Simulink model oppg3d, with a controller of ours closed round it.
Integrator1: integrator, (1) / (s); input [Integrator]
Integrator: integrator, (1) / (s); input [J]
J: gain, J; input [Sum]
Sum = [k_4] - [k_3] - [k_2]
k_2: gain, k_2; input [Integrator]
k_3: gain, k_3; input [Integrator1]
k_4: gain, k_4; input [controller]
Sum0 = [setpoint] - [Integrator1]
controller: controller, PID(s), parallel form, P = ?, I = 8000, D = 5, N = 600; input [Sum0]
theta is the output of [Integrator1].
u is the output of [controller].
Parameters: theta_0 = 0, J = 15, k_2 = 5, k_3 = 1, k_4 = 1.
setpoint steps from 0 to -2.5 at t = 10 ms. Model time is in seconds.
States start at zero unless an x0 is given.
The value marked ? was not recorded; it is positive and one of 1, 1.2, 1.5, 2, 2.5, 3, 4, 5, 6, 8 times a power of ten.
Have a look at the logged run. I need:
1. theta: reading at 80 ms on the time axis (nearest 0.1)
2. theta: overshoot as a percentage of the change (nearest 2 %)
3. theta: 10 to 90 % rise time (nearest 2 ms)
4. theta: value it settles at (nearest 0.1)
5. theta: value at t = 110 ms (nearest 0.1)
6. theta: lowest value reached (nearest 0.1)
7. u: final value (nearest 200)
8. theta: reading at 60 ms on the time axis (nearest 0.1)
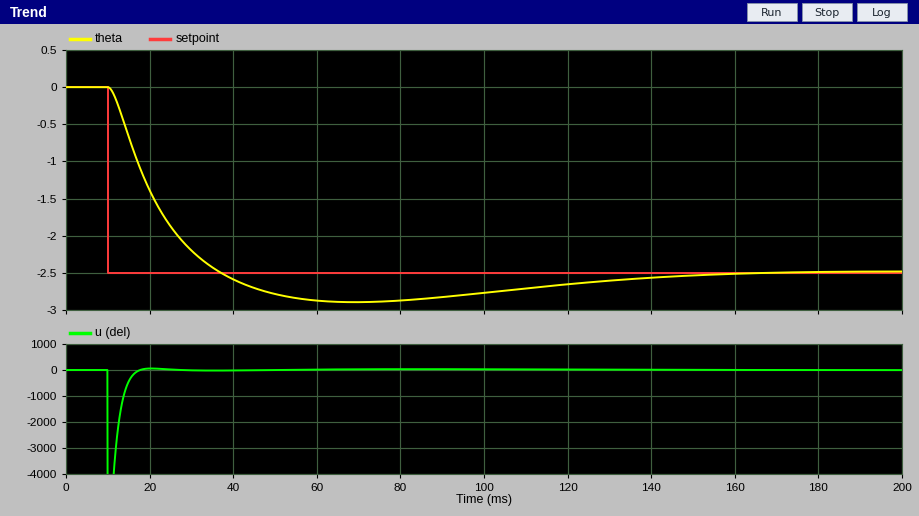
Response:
-2.9
16 %
18 ms
-2.5
-2.7
-2.9
0
-2.9
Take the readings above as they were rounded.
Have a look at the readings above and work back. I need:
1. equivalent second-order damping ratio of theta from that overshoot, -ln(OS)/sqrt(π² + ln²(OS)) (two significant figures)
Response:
0.50
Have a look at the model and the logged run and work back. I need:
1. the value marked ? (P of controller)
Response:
400
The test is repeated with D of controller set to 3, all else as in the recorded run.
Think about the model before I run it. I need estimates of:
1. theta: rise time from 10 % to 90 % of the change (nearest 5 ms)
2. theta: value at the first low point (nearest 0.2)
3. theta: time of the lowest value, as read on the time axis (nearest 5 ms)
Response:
20 ms
-3.0
60 ms
